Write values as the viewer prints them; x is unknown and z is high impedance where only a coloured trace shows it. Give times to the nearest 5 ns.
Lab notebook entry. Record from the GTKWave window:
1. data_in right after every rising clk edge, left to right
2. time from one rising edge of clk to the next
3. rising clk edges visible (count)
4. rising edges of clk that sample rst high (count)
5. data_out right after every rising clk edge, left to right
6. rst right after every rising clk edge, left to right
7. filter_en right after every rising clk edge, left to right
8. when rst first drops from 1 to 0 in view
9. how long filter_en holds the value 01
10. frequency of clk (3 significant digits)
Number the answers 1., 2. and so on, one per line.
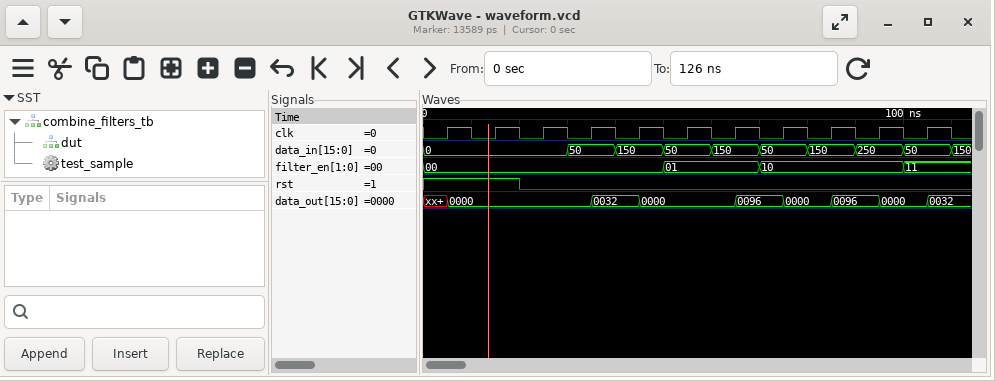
1. 0, 0, 0, 50, 150, 50, 150, 50, 150, 250, 50
2. 10 ns
3. 11
4. 2
5. 0000, 0000, 0000, 0032, 0000, 0000, 0096, 0000, 0096, 0000, 0032
6. 1 1 0 0 0 0 0 0 0 0 0
7. 00, 00, 00, 00, 00, 01, 01, 10, 10, 10, 11
8. 20 ns
9. 20 ns
10. 100 MHz
